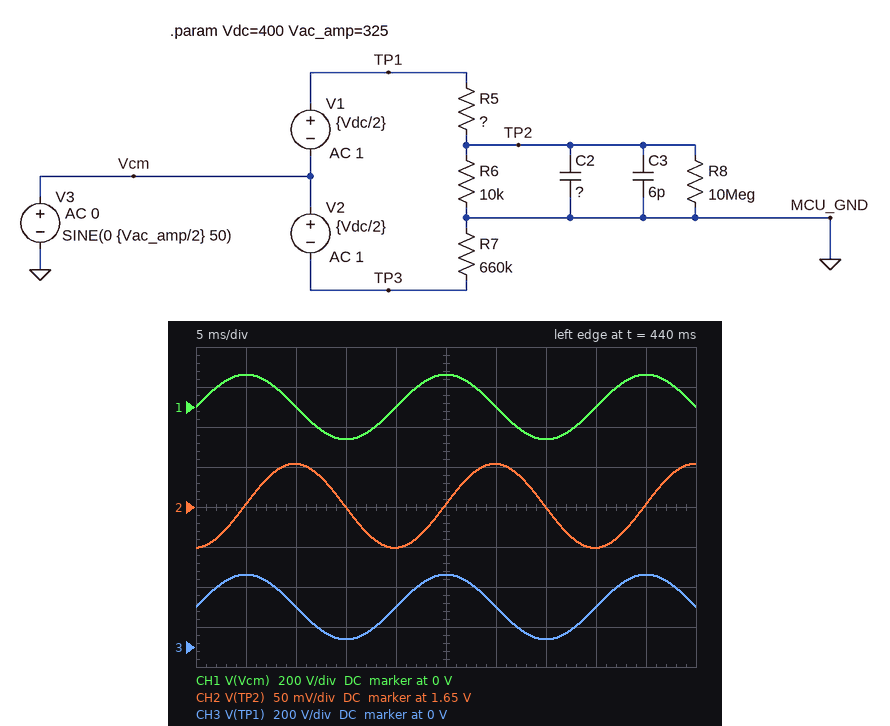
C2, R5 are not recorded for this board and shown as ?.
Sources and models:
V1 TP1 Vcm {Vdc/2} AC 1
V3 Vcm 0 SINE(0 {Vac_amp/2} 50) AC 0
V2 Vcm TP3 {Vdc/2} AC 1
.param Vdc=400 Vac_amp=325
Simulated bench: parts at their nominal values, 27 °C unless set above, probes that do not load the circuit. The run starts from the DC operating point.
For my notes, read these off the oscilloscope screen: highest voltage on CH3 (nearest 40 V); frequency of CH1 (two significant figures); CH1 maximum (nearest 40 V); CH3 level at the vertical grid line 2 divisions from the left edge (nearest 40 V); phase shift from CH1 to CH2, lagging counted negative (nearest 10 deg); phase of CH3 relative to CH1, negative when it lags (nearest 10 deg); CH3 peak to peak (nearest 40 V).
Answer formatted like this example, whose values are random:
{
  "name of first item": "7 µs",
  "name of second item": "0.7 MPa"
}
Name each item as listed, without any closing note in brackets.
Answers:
{
  "highest voltage on CH3": "360 V",
  "frequency of CH1": "50 Hz",
  "CH1 maximum": "160 V",
  "CH3 level at the vertical grid line 2 divisions from the left edge": "200 V",
  "phase shift from CH1 to CH2, lagging counted negative": "-90 deg",
  "phase of CH3 relative to CH1, negative when it lags": "0 deg",
  "CH3 peak to peak": "320 V"
}
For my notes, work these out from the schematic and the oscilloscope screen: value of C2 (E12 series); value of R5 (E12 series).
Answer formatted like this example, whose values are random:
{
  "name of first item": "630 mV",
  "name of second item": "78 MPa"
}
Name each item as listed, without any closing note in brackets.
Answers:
{
  "value of C2": "8.2 µF",
  "value of R5": "1.2 MΩ"
}
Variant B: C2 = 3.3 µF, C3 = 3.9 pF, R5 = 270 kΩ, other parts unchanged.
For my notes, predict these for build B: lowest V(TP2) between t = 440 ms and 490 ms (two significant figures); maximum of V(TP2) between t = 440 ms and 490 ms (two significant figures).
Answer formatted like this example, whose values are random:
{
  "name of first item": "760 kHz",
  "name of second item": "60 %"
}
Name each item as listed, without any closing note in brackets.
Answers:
{
  "lowest V(TP2) between t = 440 ms and 490 ms": "6.6 V",
  "maximum of V(TP2) between t = 440 ms and 490 ms": "7.7 V"
}
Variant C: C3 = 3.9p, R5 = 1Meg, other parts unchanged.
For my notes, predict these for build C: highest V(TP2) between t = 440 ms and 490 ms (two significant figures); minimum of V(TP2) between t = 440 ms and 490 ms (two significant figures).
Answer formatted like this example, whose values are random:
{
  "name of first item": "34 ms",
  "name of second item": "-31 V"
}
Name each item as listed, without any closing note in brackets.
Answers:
{
  "highest V(TP2) between t = 440 ms and 490 ms": "2.0 V",
  "minimum of V(TP2) between t = 440 ms and 490 ms": "1.9 V"
}
